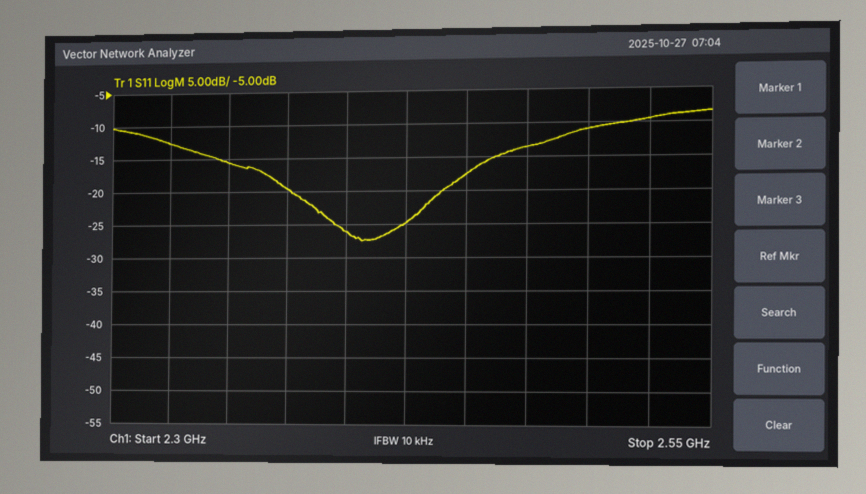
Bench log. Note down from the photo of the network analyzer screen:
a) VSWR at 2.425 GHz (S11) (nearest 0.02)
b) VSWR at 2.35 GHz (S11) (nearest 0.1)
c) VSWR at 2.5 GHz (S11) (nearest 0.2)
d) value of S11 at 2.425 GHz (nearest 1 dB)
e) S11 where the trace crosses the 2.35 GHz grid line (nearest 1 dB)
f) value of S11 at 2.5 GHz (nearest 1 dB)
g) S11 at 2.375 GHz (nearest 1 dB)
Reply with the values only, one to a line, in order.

1.12
1.4
1.8
-25 dB
-16 dB
-11 dB
-20 dB
